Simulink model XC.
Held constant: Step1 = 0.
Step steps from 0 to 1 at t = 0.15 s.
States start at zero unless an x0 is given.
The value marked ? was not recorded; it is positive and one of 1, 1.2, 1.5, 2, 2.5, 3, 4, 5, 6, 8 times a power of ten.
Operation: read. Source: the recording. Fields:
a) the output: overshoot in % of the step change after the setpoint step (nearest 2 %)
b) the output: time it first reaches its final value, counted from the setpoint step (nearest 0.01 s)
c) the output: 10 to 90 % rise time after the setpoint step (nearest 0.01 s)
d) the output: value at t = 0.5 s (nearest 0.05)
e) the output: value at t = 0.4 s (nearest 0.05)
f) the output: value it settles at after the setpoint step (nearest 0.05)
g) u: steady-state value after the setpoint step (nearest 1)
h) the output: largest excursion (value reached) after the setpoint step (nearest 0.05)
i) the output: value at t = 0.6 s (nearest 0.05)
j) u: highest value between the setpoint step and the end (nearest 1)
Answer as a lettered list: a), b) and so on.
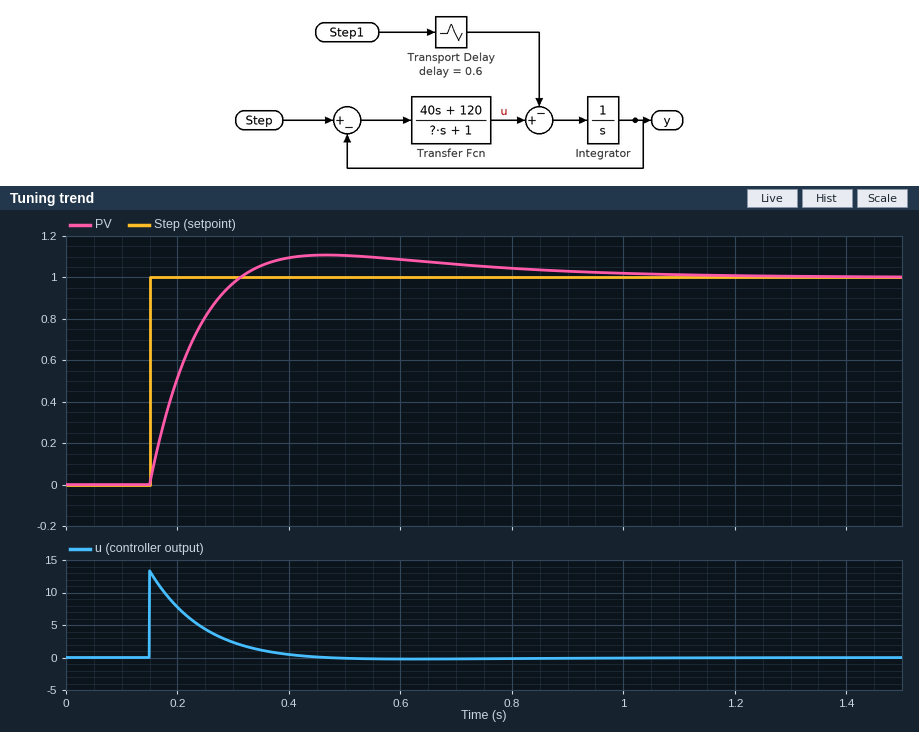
a) 10 %
b) 0.16 s
c) 0.12 s
d) 1.10
e) 1.10
f) 1.00
g) 0
h) 1.10
i) 1.10
j) 13
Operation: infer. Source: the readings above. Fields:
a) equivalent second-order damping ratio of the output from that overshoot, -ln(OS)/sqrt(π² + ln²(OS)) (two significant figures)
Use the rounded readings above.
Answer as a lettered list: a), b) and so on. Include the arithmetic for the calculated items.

a) ln(0.1) = -2.303; 2.303 / sqrt(9.870 + 5.302) = 0.59
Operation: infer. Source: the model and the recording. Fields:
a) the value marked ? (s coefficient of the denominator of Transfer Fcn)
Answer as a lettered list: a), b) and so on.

a) 3
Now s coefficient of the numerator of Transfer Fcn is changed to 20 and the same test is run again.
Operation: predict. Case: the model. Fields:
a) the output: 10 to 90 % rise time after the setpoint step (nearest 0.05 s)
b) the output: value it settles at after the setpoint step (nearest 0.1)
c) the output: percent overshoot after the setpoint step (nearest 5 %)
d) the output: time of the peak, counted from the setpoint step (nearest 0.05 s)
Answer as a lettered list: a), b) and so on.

a) 0.15 s
b) 1.0
c) 25 %
d) 0.40 s
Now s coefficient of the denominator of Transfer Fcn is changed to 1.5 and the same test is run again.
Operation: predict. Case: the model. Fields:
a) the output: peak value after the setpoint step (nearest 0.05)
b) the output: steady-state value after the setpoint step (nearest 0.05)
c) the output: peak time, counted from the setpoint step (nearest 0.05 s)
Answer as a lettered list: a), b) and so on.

a) 1.05
b) 1.00
c) 0.20 s
